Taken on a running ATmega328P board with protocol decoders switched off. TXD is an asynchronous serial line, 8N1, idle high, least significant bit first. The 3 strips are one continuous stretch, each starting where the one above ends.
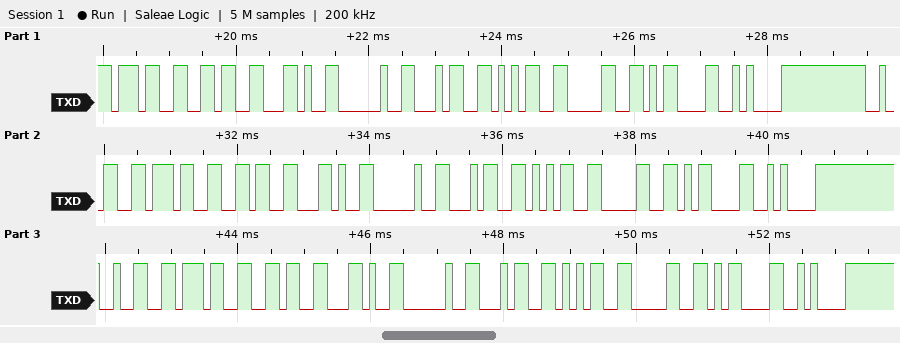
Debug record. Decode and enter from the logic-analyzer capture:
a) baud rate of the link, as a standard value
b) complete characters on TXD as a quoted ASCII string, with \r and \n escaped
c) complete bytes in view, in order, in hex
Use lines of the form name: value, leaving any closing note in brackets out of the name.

baud rate of the link, as a standard value: 9600 baud
complete characters on TXD as a quoted ASCII string, with \r and \n escaped: "76, 450\r\n276, 450\r\n276, 450\r\n"
complete bytes in view, in order, in hex: 37 36 2C 20 34 35 30 0D 0A 32 37 36 2C 20 34 35 30 0D 0A 32 37 36 2C 20 34 35 30 0D 0A
